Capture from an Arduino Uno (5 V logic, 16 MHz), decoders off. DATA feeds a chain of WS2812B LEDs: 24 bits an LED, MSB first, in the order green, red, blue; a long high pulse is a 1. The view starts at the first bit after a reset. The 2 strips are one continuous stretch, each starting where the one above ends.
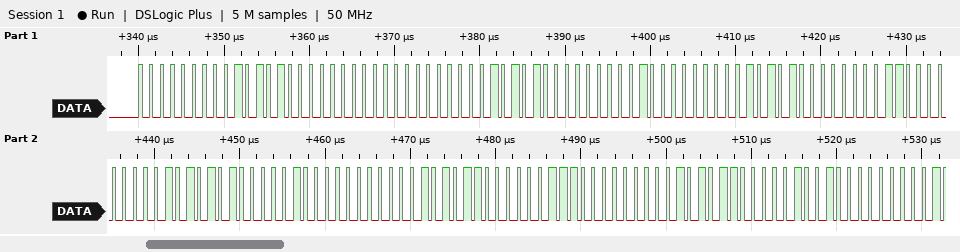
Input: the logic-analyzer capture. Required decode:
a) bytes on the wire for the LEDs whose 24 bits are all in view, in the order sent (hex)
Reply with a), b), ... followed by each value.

a) 00 54 00 00 54 01 00 54 03 00 55 04 00 56 07 00 56 09
